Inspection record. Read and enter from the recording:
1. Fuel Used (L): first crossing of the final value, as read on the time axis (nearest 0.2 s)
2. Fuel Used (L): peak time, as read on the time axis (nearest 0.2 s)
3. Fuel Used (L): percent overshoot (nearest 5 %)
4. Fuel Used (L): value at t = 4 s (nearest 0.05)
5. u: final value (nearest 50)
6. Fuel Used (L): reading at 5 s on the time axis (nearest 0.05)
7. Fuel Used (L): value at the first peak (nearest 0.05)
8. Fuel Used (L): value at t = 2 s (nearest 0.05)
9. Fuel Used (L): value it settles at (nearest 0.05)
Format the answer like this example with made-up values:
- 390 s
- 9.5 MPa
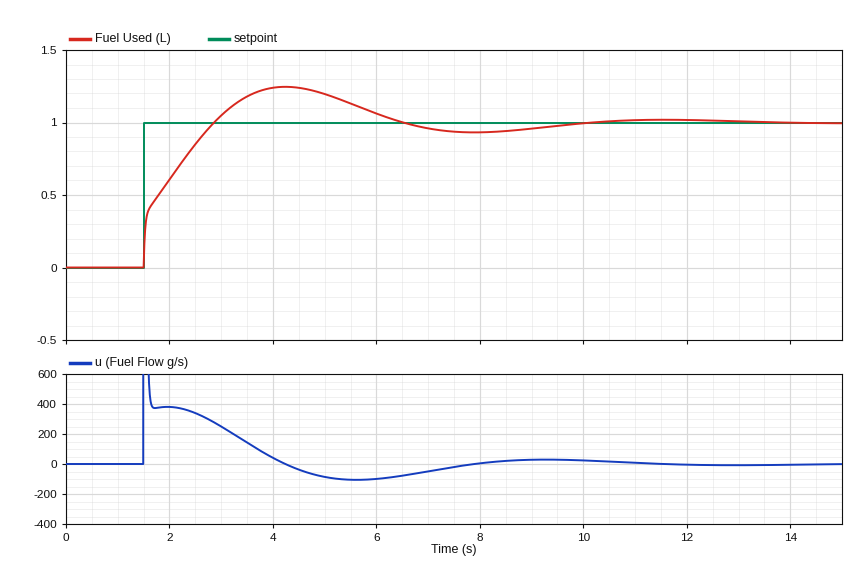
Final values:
- 2.8 s
- 4.2 s
- 25 %
- 1.25
- 0
- 1.20
- 1.25
- 0.60
- 1.00
